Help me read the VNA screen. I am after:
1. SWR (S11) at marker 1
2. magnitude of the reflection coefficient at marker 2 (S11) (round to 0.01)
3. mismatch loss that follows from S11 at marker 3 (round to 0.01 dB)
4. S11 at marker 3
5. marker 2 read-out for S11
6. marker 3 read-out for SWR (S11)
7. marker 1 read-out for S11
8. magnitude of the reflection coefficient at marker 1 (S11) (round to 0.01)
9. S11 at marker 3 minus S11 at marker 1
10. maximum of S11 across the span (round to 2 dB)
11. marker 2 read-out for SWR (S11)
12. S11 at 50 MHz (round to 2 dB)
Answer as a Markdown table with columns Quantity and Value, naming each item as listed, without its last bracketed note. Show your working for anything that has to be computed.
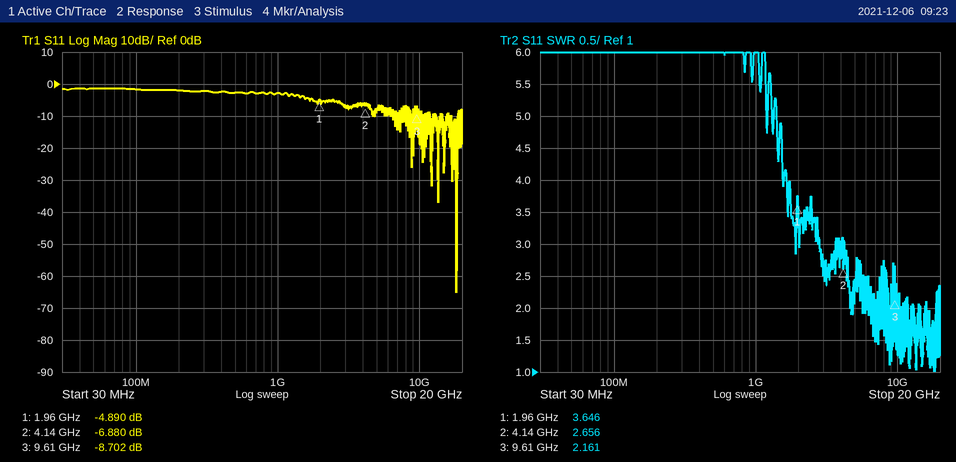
| Quantity | Value |
|---|---|
| SWR (S11) at marker 1 | 3.646 |
| magnitude of the reflection coefficient at marker 2 (S11) | 10^(-6.88/20) ≈ 0.45 |
| mismatch loss that follows from S11 at marker 3 | −10 log10(1 − 10^(-8.702/10)) ≈ 0.63 dB |
| S11 at marker 3 | -8.702 dB |
| marker 2 read-out for S11 | -6.880 dB |
| marker 3 read-out for SWR | 2.161 |
| marker 1 read-out for S11 | -4.890 dB |
| magnitude of the reflection coefficient at marker 1 (S11) | 10^(-4.89/20) ≈ 0.57 |
| S11 at marker 3 minus S11 at marker 1 | -8.702 − (-4.89) = -3.812 dB |
| maximum of S11 across the span | -2 dB |
| marker 2 read-out for SWR | 2.656 |
| S11 at 50 MHz | -2 dB |
